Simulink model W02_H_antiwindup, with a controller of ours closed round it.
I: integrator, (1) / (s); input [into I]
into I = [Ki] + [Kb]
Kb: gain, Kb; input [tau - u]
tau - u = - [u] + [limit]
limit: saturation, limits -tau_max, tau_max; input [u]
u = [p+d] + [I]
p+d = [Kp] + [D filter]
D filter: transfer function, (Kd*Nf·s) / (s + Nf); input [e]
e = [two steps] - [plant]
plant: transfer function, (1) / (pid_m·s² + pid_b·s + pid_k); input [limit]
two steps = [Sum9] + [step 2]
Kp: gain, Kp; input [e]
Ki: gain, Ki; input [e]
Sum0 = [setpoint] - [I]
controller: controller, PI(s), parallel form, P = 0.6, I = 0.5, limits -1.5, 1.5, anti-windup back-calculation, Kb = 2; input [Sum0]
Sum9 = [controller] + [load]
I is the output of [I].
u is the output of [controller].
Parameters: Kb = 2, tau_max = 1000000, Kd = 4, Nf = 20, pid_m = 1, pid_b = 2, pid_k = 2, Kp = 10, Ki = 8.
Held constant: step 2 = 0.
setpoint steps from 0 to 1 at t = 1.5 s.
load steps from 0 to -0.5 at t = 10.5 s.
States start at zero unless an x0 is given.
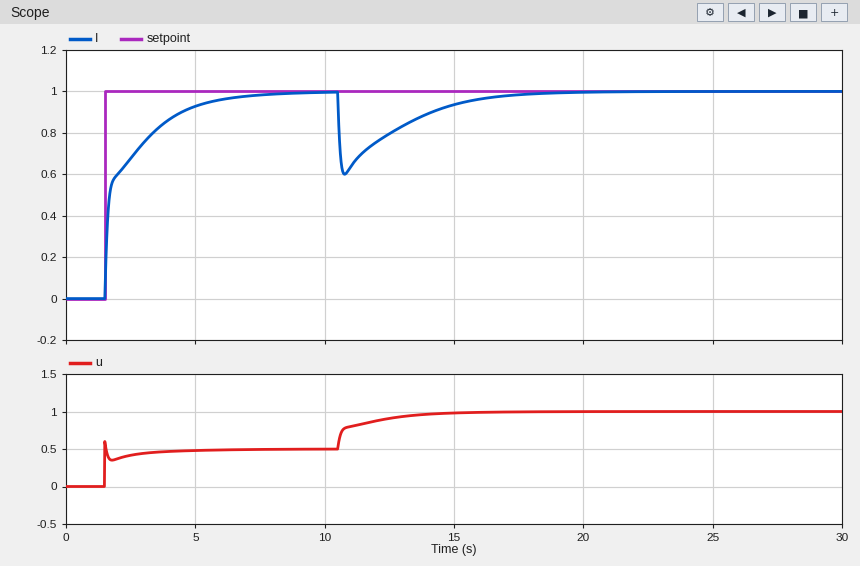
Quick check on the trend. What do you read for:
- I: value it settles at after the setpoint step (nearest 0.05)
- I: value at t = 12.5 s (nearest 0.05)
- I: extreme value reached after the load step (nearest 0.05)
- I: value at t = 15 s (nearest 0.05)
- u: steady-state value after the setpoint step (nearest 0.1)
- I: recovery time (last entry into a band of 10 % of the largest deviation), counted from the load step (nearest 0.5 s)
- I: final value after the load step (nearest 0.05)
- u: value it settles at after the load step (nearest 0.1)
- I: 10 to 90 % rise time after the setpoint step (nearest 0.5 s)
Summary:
1.00
0.80
0.60
0.95
0.5
5.5 s
1.00
1.0
3.0 s
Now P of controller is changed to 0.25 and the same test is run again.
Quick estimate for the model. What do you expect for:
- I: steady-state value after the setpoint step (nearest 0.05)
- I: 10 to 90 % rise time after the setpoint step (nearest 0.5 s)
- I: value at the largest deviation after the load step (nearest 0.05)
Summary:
1.00
2.5 s
0.45
